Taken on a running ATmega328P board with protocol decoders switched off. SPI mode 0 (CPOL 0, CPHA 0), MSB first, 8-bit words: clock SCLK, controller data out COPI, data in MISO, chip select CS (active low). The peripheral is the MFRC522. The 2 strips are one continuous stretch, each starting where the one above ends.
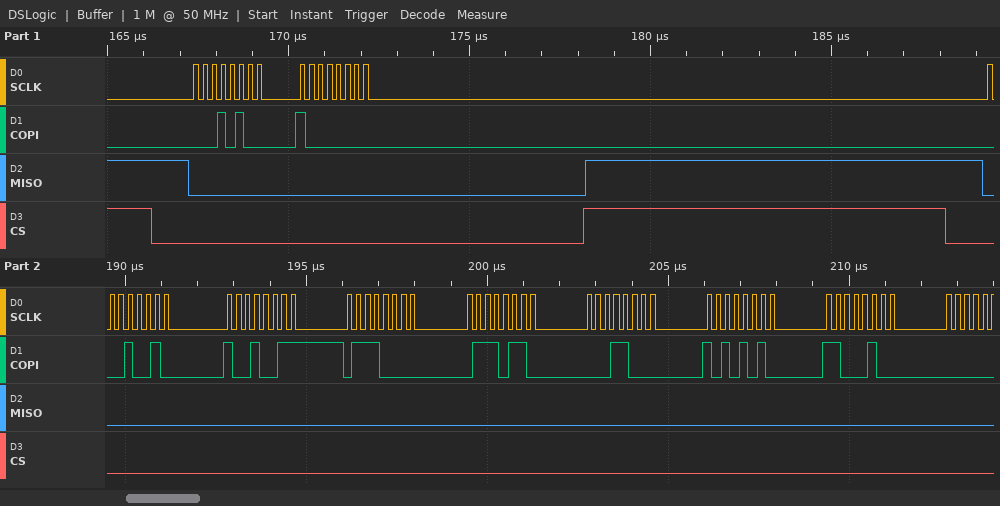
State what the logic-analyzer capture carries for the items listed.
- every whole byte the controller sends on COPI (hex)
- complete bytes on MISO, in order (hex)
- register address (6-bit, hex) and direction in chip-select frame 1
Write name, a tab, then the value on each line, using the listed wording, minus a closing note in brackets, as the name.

every whole byte the controller sends on COPI	14 80 12 93 70 76 18 AA C4
complete bytes on MISO, in order	00 00 00 00 00 00 00 00 00
register address (6-bit, hex) and direction in chip-select frame 1	0x0A write
